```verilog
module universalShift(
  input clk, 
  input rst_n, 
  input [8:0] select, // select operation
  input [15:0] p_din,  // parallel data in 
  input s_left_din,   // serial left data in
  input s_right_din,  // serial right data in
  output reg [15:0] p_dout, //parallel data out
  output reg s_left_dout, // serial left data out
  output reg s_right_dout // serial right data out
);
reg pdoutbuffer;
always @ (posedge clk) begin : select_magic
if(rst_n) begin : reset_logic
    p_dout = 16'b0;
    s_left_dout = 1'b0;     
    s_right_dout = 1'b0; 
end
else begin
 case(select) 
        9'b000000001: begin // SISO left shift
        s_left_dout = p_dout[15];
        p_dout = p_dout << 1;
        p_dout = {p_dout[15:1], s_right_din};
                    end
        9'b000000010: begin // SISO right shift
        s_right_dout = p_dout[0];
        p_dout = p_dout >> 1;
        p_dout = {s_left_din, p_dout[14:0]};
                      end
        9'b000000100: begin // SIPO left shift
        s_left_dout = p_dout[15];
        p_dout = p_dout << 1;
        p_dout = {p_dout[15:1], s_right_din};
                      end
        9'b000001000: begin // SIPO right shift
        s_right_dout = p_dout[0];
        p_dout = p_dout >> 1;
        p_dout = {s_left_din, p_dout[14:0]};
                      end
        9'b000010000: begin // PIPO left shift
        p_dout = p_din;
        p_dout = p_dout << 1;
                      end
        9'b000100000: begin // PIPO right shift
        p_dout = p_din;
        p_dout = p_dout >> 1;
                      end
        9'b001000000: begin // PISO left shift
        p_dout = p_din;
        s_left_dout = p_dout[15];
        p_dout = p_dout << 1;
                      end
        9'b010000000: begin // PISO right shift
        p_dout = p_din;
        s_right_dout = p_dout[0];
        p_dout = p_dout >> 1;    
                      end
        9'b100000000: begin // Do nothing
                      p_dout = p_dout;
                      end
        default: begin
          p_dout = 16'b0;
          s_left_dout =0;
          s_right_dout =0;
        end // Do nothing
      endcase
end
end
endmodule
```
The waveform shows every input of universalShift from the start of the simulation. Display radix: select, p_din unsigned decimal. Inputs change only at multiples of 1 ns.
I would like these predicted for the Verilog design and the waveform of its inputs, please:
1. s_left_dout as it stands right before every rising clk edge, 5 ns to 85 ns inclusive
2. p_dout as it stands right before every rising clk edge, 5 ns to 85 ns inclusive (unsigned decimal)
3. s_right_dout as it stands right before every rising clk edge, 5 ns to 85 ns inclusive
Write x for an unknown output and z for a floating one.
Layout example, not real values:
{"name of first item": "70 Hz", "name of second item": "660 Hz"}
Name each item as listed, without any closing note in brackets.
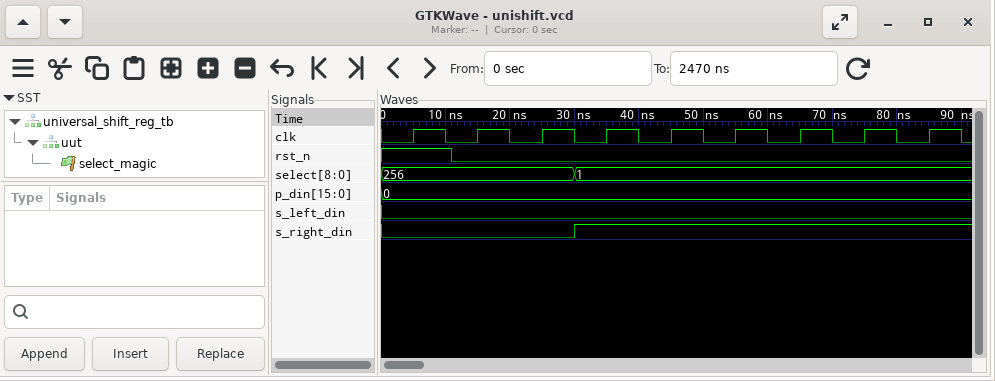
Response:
{"s_left_dout as it stands right before every rising clk edge, 5 ns to 85 ns inclusive": "x 0 0 0 0 0 0 0 0", "p_dout as it stands right before every rising clk edge, 5 ns to 85 ns inclusive": "x, 0, 0, 0, 1, 3, 7, 15, 31", "s_right_dout as it stands right before every rising clk edge, 5 ns to 85 ns inclusive": "x 0 0 0 0 0 0 0 0"}
